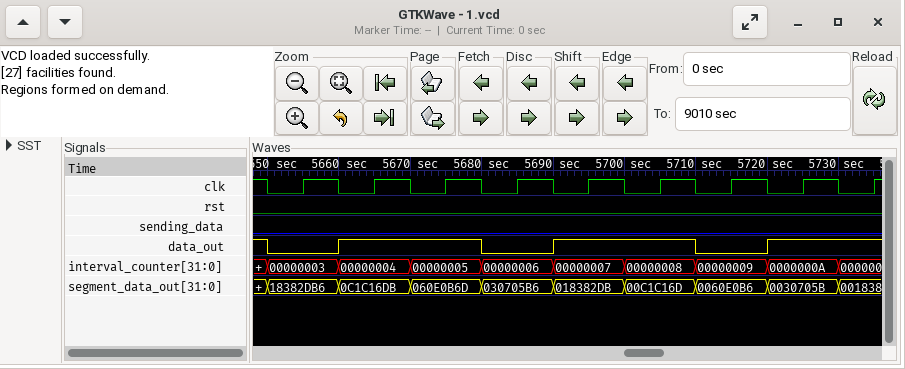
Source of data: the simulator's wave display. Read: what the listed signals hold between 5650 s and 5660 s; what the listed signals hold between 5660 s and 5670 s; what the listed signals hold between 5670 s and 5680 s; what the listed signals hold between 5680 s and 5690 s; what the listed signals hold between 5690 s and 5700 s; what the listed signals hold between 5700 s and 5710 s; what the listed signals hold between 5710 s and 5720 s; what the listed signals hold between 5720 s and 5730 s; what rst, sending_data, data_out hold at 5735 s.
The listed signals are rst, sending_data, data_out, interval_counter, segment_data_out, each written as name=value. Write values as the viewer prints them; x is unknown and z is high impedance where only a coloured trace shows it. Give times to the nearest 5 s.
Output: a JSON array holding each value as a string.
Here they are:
["rst=0, sending_data=0, data_out=0, interval_counter=00000003, segment_data_out=18382DB6", "rst=0, sending_data=0, data_out=1, interval_counter=00000004, segment_data_out=0C1C16DB", "rst=0, sending_data=0, data_out=1, interval_counter=00000005, segment_data_out=060E0B6D", "rst=0, sending_data=0, data_out=0, interval_counter=00000006, segment_data_out=030705B6", "rst=0, sending_data=0, data_out=1, interval_counter=00000007, segment_data_out=018382DB", "rst=0, sending_data=0, data_out=1, interval_counter=00000008, segment_data_out=00C1C16D", "rst=0, sending_data=0, data_out=0, interval_counter=00000009, segment_data_out=0060E0B6", "rst=0, sending_data=0, data_out=1, interval_counter=0000000A, segment_data_out=0030705B", "rst=0, sending_data=0, data_out=1"]
